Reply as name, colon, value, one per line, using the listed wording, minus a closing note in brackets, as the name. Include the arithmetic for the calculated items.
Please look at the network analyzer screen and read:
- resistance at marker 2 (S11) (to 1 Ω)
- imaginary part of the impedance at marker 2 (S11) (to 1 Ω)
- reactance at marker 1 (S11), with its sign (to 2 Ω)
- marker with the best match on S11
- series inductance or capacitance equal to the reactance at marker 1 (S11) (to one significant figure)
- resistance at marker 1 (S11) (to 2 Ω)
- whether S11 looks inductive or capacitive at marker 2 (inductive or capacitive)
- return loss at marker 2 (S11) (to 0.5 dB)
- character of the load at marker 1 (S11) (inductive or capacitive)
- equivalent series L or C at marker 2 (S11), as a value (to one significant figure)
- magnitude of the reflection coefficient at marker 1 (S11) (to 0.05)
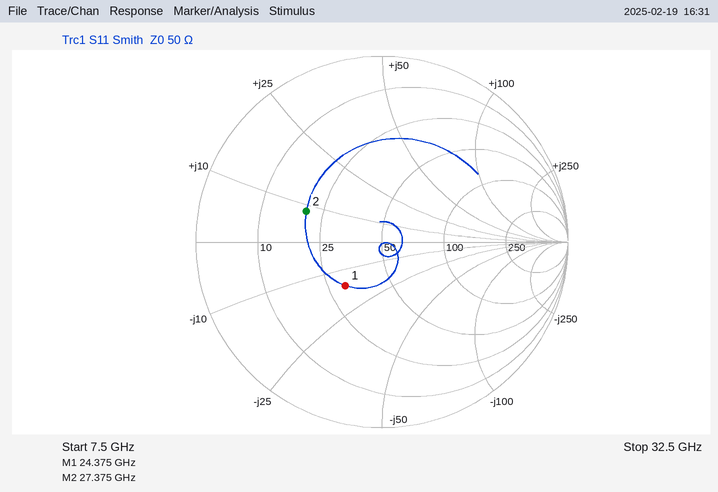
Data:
resistance at marker 2 (S11): 20 Ω
imaginary part of the impedance at marker 2 (S11): +8 Ω
reactance at marker 1 (S11), with its sign: -16 Ω
marker with the best match on S11: marker 1
series inductance or capacitance equal to the reactance at marker 1 (S11): C = 1/(2π × 24.375 GHz × 16 Ω) ≈ 408 fF, so 400 fF to one significant figure
resistance at marker 1 (S11): 30 Ω
whether S11 looks inductive or capacitive at marker 2: inductive
return loss at marker 2 (S11): 7.0 dB
character of the load at marker 1 (S11): capacitive
equivalent series L or C at marker 2 (S11), as a value: L = 8 Ω/(2π × 27.375 GHz) ≈ 46.5 pH, so 50 pH to one significant figure
magnitude of the reflection coefficient at marker 1 (S11): 0.30
